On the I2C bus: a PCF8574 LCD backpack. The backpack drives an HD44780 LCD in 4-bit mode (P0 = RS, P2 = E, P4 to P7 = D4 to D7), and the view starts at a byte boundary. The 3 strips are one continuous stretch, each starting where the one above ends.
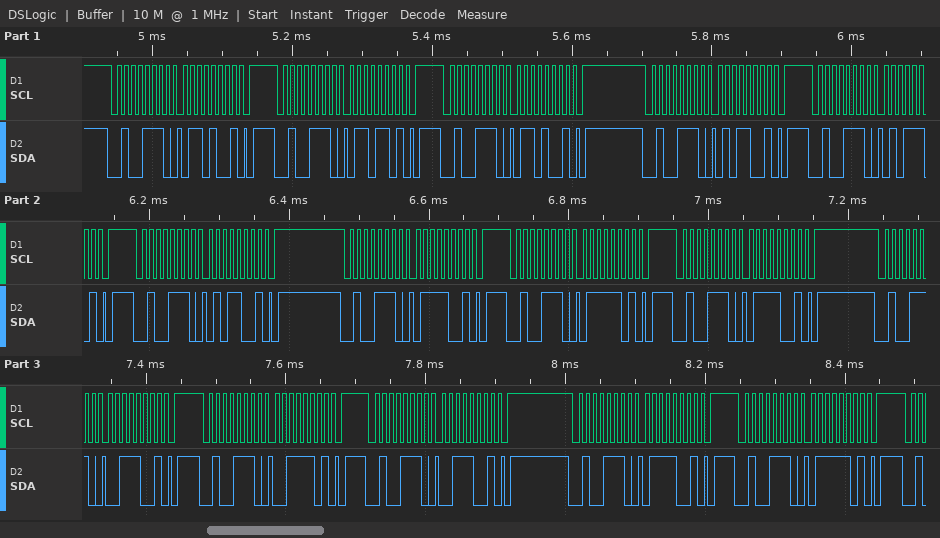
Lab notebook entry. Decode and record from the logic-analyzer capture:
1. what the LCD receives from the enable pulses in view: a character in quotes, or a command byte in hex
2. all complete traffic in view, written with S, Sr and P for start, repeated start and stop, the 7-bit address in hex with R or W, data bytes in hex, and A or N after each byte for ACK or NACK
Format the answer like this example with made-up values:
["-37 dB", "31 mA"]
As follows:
["'e' 's'", "S 27W A 69 A P S 27W A 6D A P S 27W A 69 A P S 27W A 59 A P S 27W A 5D A P S 27W A 59 A P S 27W A 79 A P S 27W A 7D A P S 27W A 79 A P S 27W A 39 A P S 27W A 3D A P S 27W A 39 A P S 27W A 79 A P S 27W A 7D A P"]
